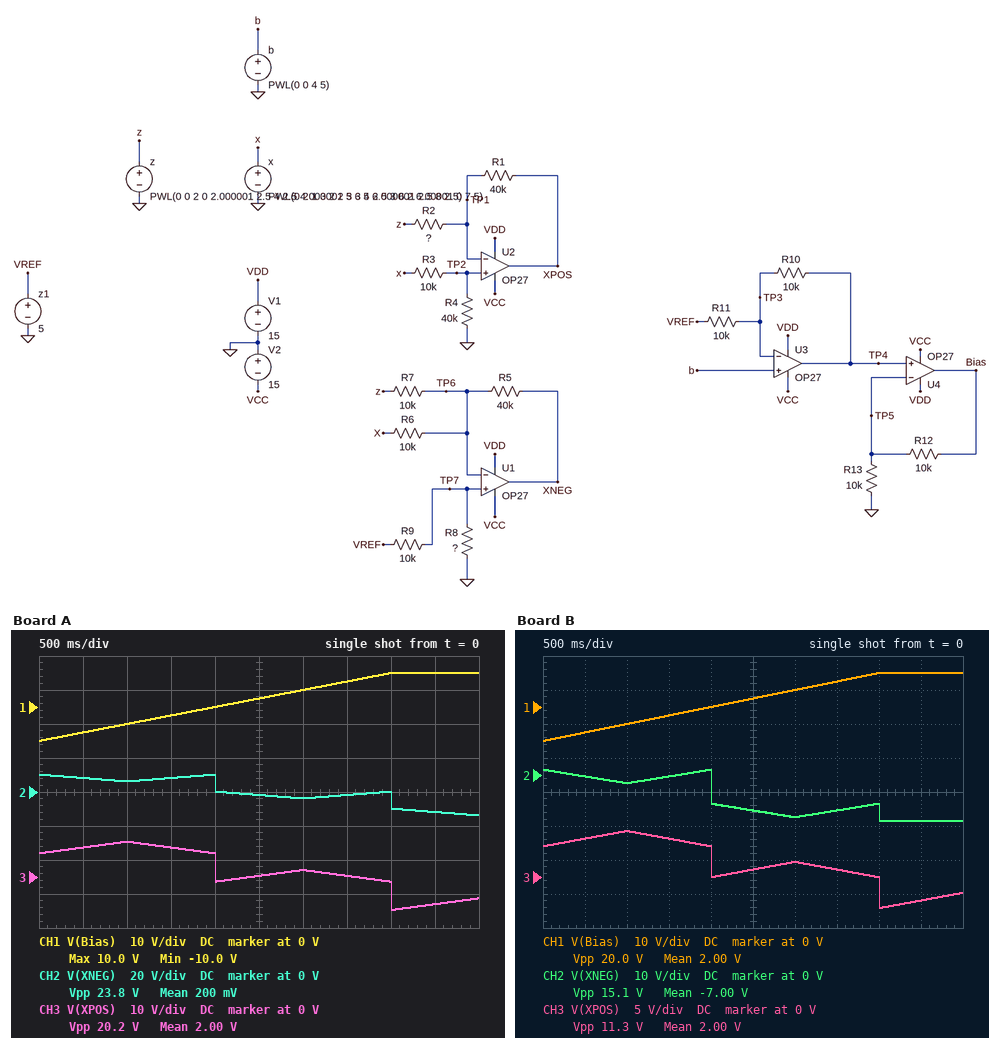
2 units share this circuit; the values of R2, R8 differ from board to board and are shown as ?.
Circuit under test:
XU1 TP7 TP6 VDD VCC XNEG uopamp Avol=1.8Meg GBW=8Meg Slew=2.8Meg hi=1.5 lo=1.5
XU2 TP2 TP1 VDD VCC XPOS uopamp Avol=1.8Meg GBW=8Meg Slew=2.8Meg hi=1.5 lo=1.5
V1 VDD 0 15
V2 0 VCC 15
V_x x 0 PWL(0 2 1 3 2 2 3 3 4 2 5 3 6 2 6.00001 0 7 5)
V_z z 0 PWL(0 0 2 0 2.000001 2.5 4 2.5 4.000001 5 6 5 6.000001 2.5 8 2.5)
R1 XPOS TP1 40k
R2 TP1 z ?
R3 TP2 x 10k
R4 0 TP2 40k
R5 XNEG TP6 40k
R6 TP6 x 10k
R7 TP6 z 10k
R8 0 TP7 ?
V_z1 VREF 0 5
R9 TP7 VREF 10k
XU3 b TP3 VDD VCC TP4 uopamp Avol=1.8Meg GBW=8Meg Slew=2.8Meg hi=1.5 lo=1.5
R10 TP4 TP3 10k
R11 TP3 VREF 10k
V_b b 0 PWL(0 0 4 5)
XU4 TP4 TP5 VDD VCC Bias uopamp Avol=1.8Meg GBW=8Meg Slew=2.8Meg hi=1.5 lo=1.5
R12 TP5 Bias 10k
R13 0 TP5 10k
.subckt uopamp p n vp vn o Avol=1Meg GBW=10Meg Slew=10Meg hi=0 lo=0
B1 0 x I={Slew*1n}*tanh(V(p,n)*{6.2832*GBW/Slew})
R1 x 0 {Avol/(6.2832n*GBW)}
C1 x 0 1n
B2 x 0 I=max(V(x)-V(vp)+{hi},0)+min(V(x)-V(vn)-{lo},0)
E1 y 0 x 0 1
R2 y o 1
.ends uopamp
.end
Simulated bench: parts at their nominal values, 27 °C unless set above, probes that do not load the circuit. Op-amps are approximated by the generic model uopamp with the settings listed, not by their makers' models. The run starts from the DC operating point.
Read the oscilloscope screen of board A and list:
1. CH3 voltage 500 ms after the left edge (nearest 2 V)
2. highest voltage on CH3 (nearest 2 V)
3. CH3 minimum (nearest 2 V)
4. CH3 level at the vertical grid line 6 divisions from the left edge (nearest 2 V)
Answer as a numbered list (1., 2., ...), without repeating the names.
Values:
1. 8 V
2. 10 V
3. -10 V
4. 2 V
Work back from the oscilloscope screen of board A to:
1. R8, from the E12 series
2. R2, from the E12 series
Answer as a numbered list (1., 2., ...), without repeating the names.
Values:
1. 6.8 kΩ
2. 12 kΩ
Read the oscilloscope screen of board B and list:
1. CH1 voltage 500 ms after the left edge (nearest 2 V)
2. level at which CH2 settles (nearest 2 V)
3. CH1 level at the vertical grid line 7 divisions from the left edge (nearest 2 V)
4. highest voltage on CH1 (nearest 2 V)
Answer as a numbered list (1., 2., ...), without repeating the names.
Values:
1. -8 V
2. -14 V
3. 8 V
4. 10 V
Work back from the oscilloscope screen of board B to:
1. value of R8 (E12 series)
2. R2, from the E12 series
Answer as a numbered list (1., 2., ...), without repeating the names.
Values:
1. 2.7 kΩ
2. 22 kΩ
